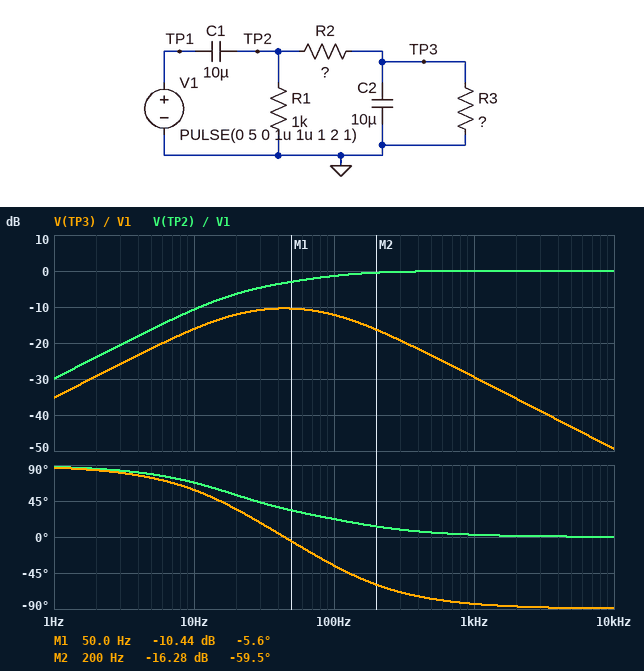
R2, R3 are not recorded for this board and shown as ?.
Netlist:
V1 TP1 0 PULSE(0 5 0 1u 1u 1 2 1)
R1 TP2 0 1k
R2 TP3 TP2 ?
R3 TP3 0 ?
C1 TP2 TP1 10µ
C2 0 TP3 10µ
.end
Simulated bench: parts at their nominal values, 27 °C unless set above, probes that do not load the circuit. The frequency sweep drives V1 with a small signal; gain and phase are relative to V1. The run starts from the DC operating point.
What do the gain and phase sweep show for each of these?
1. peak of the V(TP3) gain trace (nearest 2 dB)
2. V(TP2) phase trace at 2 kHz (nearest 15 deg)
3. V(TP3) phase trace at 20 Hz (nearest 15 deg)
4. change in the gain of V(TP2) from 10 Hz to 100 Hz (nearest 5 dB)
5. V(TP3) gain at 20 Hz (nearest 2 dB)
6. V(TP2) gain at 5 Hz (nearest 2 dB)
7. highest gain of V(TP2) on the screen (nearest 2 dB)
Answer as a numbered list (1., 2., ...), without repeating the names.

1. -10 dB
2. 0 deg
3. 30 deg
4. 10 dB
5. -12 dB
6. -16 dB
7. 0 dB
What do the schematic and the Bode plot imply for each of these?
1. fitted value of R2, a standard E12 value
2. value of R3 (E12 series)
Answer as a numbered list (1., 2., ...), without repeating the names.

1. 470 Ω
2. 560 Ω
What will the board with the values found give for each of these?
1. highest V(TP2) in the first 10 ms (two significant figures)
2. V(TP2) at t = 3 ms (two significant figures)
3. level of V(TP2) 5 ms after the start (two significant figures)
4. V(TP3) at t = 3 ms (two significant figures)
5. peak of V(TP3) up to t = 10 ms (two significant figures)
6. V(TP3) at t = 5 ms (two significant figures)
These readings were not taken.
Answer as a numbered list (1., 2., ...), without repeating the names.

1. 5.0 V
2. 2.3 V
3. 1.6 V
4. 1.2 V
5. 1.2 V
6. 1.1 V
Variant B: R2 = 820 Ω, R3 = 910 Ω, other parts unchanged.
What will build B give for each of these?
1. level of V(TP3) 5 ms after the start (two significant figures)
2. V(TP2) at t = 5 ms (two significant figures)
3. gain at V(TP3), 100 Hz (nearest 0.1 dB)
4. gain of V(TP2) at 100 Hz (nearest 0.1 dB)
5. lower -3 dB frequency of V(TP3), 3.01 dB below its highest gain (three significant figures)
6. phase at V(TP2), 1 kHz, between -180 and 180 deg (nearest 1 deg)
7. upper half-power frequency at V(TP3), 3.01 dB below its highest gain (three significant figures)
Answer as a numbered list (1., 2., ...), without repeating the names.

1. 1.0 V
2. 2.0 V
3. -15.5 dB
4. -0.7 dB
5. 11.1 Hz
6. 2 deg
7. 83.3 Hz
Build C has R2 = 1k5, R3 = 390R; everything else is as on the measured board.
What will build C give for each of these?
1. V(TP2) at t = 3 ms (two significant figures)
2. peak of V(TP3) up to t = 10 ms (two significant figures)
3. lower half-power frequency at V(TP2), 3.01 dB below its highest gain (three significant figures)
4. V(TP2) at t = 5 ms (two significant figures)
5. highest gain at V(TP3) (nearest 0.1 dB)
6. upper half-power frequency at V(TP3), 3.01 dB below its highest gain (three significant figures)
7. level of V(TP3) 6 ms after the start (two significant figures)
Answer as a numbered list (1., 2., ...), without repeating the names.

1. 3.1 V
2. 520 mV
3. 25.7 Hz
4. 2.3 V
5. -17.3 dB
6. 91.6 Hz
7. 490 mV
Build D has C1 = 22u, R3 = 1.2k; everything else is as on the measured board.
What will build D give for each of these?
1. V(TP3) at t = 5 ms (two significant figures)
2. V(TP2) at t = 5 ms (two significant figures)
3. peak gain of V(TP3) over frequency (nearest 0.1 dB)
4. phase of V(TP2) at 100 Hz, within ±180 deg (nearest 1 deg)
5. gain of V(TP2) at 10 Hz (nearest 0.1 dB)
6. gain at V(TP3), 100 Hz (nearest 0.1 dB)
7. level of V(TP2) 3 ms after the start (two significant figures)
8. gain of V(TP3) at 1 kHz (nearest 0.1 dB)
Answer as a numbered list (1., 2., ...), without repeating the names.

1. 2.0 V
2. 3.0 V
3. -6.3 dB
4. 11 deg
5. -4.7 dB
6. -10.8 dB
7. 3.5 V
8. -29.4 dB
